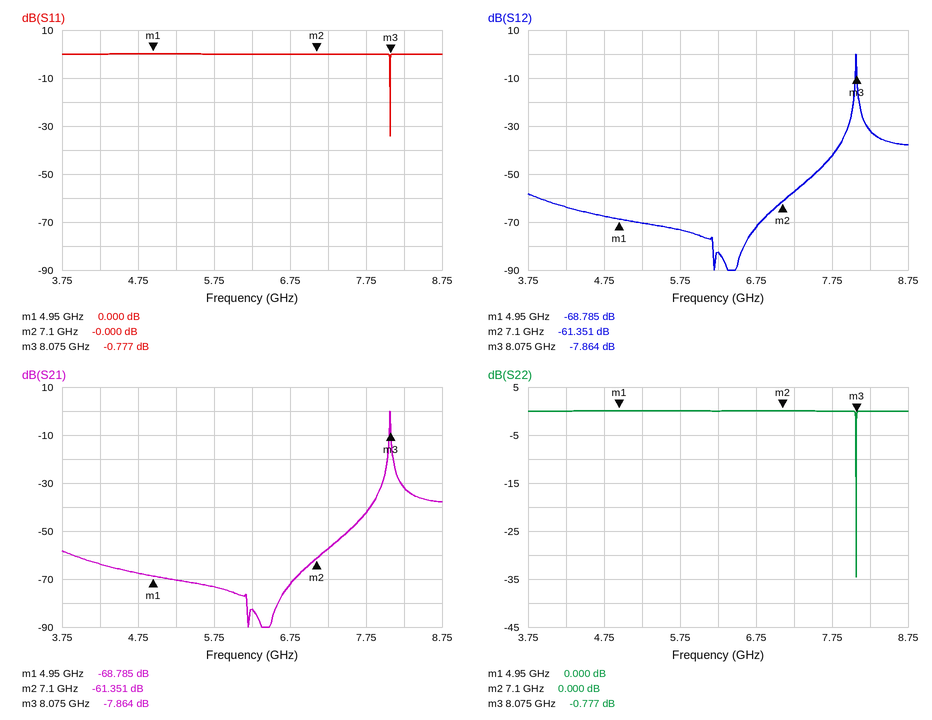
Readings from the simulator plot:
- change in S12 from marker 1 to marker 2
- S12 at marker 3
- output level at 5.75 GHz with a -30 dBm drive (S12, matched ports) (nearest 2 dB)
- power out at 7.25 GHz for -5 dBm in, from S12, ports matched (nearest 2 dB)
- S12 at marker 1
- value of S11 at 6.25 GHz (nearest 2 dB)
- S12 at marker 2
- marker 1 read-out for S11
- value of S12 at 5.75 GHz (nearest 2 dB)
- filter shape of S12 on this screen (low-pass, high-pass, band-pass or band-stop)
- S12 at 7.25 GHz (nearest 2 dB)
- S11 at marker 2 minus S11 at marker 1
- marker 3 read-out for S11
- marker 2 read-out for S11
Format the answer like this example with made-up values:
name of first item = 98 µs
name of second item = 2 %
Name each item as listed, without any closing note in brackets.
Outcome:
change in S12 from marker 1 to marker 2 = 7.434 dB
S12 at marker 3 = -7.864 dB
output level at 5.75 GHz with a -30 dBm drive (S12, matched ports) = -104 dBm
power out at 7.25 GHz for -5 dBm in, from S12, ports matched = -62 dBm
S12 at marker 1 = -68.785 dB
value of S11 at 6.25 GHz = 0 dB
S12 at marker 2 = -61.351 dB
marker 1 read-out for S11 = 0.000 dB
value of S12 at 5.75 GHz = -74 dB
filter shape of S12 on this screen = band-pass
S12 at 7.25 GHz = -58 dB
S11 at marker 2 minus S11 at marker 1 = 0.000 dB
marker 3 read-out for S11 = -0.777 dB
marker 2 read-out for S11 = -0.000 dB
